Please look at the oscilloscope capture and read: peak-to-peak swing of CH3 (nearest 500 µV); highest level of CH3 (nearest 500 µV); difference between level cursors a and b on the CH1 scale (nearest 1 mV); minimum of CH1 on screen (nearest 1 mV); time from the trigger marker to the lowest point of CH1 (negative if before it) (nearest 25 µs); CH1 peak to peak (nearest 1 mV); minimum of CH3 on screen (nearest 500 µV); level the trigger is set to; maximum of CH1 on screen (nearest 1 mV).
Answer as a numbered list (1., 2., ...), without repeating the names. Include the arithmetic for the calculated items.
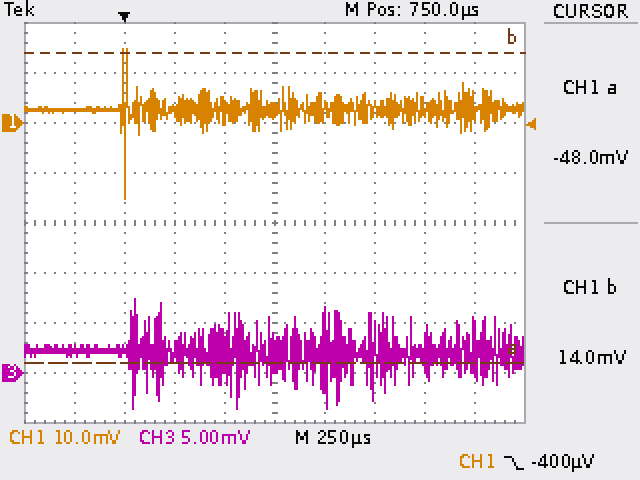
1. 7.5 mV − (-3.5 mV) = 11.0 mV
2. 7.5 mV
3. 62 mV
4. -15 mV
5. 0 µs
6. 15 mV − (-15 mV) = 30 mV
7. -3.5 mV
8. -400 µV
9. 15 mV
